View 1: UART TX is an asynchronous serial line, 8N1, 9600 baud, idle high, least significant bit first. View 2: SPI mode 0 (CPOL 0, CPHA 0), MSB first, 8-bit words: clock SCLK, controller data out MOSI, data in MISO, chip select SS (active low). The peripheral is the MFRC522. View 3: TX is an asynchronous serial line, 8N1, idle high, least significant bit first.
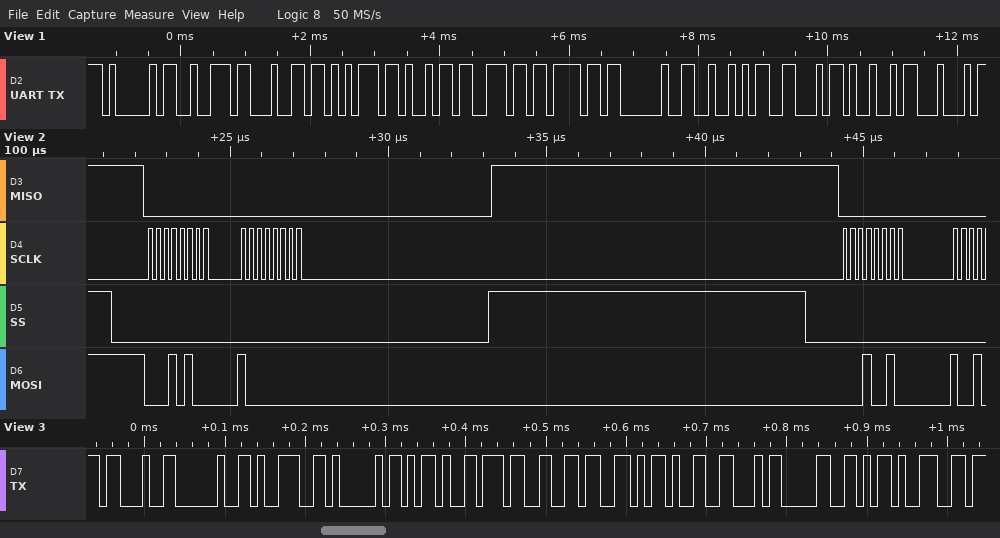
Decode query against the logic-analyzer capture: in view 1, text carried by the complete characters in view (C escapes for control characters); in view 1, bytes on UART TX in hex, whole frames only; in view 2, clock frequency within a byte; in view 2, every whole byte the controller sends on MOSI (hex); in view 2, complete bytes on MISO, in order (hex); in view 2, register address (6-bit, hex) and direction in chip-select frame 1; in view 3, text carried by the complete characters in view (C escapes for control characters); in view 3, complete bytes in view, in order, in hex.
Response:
"Arduino RFID"
0x41 0x72 0x64 0x75 0x69 0x6E 0x6F 0x20 0x52 0x46 0x49 0x44
4 MHz
14 80 12
00 00 00
0x0A write
"# 9A-76-F0-"
23 20 39 41 2D 37 36 2D 46 30 2D
